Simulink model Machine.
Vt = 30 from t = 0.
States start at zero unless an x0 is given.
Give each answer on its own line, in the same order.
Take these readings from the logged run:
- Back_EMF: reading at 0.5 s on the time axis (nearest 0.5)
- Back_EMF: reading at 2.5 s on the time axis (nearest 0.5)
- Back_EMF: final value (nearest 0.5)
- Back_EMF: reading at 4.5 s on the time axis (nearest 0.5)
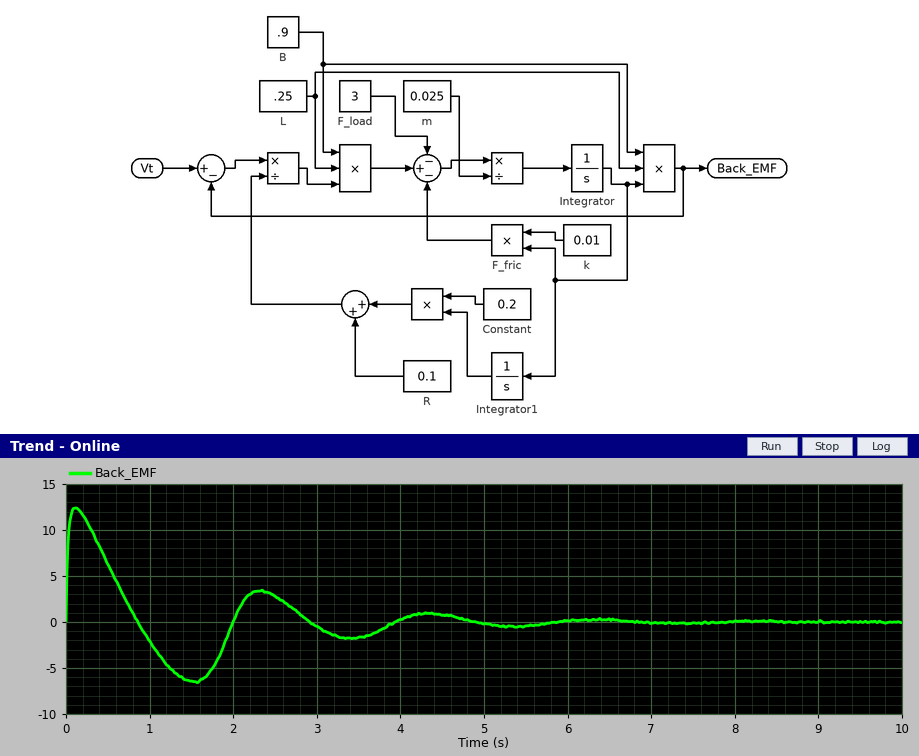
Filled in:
6.5
3.0
0.0
1.0
